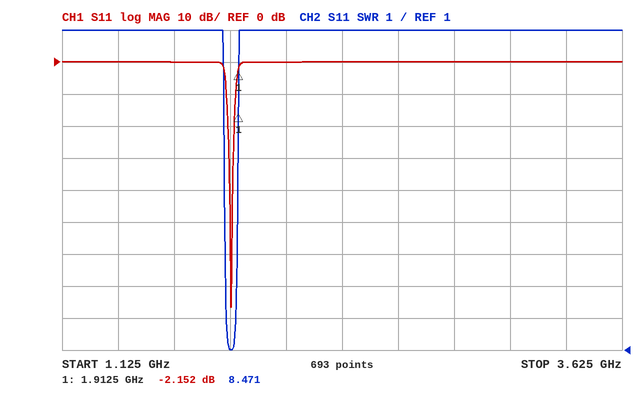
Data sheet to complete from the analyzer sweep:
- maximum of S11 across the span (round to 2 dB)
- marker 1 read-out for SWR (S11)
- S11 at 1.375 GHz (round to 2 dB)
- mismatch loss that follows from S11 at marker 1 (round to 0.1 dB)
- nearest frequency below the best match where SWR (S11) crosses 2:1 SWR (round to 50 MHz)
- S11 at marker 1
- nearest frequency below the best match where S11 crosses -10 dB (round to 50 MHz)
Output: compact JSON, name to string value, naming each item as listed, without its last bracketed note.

{"maximum of S11 across the span": "0 dB", "marker 1 read-out for SWR": "8.471", "S11 at 1.375 GHz": "0 dB", "mismatch loss that follows from S11 at marker 1": "4.1 dB", "nearest frequency below the best match where SWR (S11) crosses 2:1 SWR": "1.85 GHz", "S11 at marker 1": "-2.152 dB", "nearest frequency below the best match where S11 crosses -10 dB": "1.85 GHz"}
